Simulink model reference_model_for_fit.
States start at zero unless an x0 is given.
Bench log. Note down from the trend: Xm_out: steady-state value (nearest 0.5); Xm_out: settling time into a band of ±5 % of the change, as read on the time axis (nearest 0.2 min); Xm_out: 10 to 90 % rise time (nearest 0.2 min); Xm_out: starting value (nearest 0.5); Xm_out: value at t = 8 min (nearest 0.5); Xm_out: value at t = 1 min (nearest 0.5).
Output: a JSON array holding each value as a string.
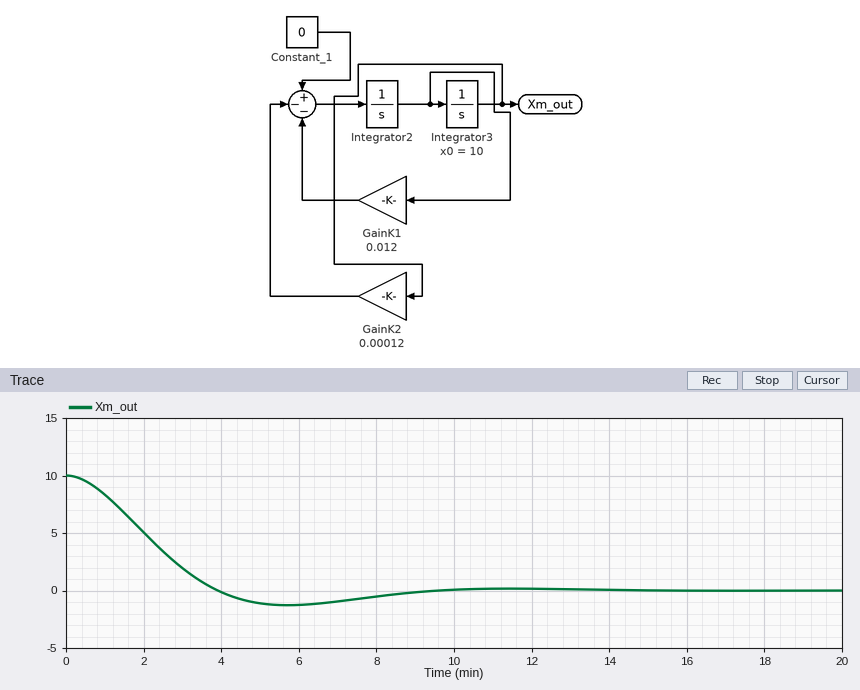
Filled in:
["0.0", "8.0 min", "2.6 min", "10.0", "-0.5", "8.5"]
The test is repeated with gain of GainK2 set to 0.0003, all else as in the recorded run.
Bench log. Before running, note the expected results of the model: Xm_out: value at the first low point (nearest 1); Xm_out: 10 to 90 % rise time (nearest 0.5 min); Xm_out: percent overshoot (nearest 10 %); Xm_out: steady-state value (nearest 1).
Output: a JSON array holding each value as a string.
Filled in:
["-3", "1.5 min", "30 %", "0"]
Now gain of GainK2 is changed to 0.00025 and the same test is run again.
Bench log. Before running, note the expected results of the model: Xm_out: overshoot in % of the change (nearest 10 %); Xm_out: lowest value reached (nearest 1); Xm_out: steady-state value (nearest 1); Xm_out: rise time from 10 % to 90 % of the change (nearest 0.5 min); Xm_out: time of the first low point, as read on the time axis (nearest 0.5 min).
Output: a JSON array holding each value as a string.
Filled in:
["30 %", "-3", "0", "1.5 min", "3.5 min"]
